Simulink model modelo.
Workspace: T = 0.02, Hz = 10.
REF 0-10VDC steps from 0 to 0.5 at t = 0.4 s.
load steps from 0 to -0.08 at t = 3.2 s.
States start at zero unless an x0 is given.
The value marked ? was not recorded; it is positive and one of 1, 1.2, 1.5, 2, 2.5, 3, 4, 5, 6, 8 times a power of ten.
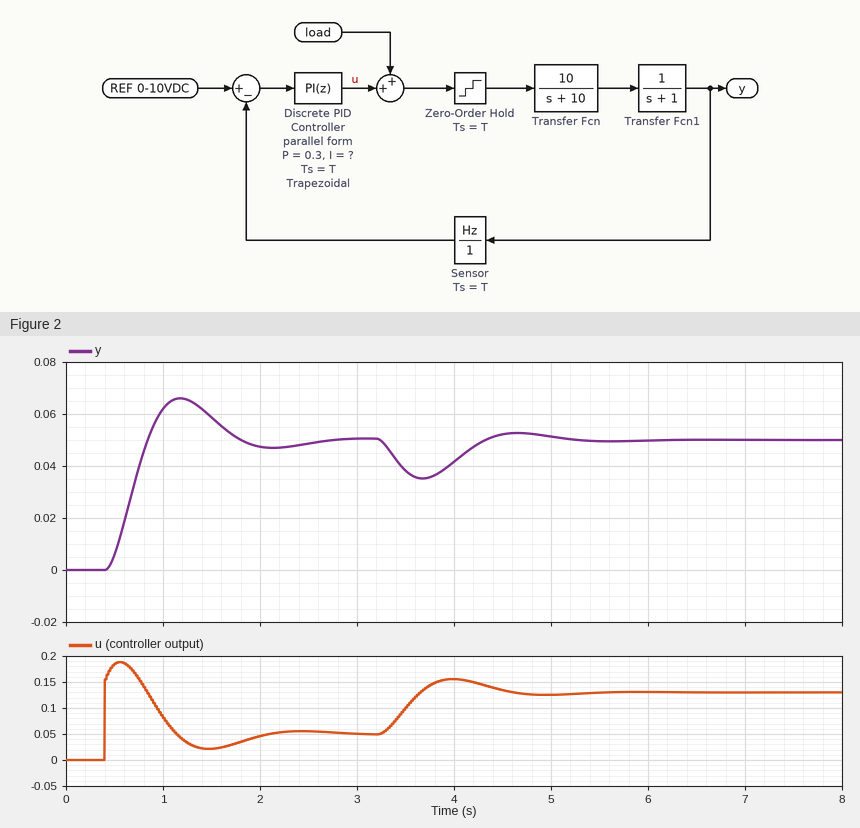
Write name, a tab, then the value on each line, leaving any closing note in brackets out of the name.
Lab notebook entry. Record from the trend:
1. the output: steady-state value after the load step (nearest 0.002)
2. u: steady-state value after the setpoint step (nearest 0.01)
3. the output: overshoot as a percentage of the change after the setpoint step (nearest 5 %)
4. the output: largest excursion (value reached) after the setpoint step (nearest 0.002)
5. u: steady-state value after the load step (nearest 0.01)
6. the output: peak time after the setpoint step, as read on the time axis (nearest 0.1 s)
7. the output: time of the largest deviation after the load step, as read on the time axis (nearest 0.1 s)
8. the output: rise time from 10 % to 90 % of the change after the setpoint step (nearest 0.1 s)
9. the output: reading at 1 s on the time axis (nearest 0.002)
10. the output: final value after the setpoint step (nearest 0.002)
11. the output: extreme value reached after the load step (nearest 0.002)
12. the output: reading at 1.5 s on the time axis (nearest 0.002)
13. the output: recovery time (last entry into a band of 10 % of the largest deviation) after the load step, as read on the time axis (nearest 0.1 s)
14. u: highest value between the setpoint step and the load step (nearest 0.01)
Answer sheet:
the output: steady-state value after the load step	0.050
u: steady-state value after the setpoint step	0.05
the output: overshoot as a percentage of the change after the setpoint step	30 %
the output: largest excursion (value reached) after the setpoint step	0.066
u: steady-state value after the load step	0.13
the output: peak time after the setpoint step, as read on the time axis	1.2 s
the output: time of the largest deviation after the load step, as read on the time axis	3.7 s
the output: rise time from 10 % to 90 % of the change after the setpoint step	0.3 s
the output: reading at 1 s on the time axis	0.062
the output: final value after the setpoint step	0.050
the output: extreme value reached after the load step	0.036
the output: reading at 1.5 s on the time axis	0.058
the output: recovery time (last entry into a band of 10 % of the largest deviation) after the load step, as read on the time axis	5.0 s
u: highest value between the setpoint step and the load step	0.19
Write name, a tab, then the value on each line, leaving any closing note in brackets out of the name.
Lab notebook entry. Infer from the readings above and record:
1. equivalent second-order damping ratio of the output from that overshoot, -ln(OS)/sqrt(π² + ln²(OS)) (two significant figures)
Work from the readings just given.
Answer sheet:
equivalent second-order damping ratio of the output from that overshoot, -ln(OS)/sqrt(π² + ln²(OS))	0.36
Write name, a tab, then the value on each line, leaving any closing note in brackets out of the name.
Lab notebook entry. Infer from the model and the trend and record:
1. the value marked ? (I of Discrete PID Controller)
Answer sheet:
the value marked ?	1
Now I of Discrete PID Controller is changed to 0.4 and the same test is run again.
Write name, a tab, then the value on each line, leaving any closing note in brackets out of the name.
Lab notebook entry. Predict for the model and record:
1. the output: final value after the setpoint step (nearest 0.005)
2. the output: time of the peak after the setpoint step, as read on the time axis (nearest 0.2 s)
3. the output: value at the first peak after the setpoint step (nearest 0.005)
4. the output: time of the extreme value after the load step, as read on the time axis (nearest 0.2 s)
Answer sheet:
the output: final value after the setpoint step	0.050
the output: time of the peak after the setpoint step, as read on the time axis	1.4 s
the output: value at the first peak after the setpoint step	0.055
the output: time of the extreme value after the load step, as read on the time axis	3.8 s
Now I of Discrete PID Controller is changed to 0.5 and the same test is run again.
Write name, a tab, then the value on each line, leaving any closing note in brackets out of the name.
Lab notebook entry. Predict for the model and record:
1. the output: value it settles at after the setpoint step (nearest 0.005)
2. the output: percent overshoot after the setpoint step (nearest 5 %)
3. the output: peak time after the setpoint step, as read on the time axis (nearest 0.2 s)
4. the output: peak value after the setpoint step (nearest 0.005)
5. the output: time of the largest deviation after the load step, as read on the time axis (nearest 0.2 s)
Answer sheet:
the output: value it settles at after the setpoint step	0.050
the output: percent overshoot after the setpoint step	10 %
the output: peak time after the setpoint step, as read on the time axis	1.4 s
the output: peak value after the setpoint step	0.055
the output: time of the largest deviation after the load step, as read on the time axis	3.8 s
